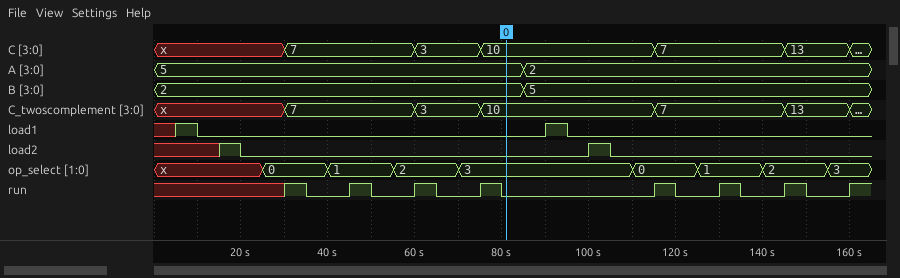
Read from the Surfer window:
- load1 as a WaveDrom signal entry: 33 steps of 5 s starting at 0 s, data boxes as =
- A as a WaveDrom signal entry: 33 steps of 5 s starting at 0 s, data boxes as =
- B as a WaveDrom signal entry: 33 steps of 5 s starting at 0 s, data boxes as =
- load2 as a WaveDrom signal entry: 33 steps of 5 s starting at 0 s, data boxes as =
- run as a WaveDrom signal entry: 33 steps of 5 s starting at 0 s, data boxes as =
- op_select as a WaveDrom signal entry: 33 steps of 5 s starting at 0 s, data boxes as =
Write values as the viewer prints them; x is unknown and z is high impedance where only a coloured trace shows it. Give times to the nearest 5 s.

{name: 'load1', wave: 'x10...............10.............'}
{name: 'A', wave: '=................=...............', data: '5 2'}
{name: 'B', wave: '=................=...............', data: '2 5'}
{name: 'load2', wave: 'x..10...............10...........'}
{name: 'run', wave: 'x.....10.10.10.10......10.10.10.1'}
{name: 'op_select', wave: 'x....=..=..=..=.......=..=..=..=.', data: '0 1 2 3 0 1 2 3'}
